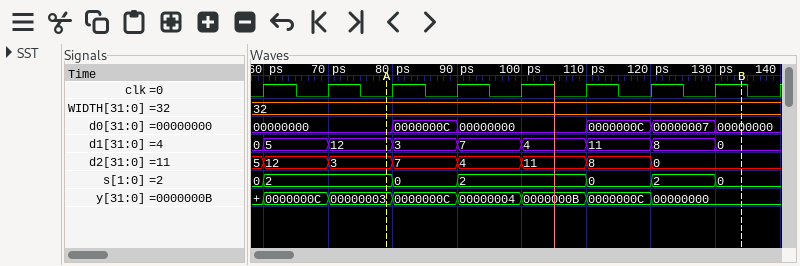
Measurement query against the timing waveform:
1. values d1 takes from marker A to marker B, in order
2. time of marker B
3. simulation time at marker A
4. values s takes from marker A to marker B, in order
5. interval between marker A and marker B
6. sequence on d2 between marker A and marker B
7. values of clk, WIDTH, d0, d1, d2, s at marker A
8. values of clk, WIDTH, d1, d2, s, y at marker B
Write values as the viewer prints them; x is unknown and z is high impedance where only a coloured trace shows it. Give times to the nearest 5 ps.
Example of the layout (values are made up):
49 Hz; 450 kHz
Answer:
12, 3, 7, 4, 11, 8, 0; 135 ps; 80 ps; 2, 0, 2, 0, 2, 0; 55 ps; 3, 7, 4, 11, 8, 0; clk=0, WIDTH=32, d0=00000000, d1=12, d2=3, s=2; clk=1, WIDTH=32, d1=0, d2=0, s=0, y=00000000
